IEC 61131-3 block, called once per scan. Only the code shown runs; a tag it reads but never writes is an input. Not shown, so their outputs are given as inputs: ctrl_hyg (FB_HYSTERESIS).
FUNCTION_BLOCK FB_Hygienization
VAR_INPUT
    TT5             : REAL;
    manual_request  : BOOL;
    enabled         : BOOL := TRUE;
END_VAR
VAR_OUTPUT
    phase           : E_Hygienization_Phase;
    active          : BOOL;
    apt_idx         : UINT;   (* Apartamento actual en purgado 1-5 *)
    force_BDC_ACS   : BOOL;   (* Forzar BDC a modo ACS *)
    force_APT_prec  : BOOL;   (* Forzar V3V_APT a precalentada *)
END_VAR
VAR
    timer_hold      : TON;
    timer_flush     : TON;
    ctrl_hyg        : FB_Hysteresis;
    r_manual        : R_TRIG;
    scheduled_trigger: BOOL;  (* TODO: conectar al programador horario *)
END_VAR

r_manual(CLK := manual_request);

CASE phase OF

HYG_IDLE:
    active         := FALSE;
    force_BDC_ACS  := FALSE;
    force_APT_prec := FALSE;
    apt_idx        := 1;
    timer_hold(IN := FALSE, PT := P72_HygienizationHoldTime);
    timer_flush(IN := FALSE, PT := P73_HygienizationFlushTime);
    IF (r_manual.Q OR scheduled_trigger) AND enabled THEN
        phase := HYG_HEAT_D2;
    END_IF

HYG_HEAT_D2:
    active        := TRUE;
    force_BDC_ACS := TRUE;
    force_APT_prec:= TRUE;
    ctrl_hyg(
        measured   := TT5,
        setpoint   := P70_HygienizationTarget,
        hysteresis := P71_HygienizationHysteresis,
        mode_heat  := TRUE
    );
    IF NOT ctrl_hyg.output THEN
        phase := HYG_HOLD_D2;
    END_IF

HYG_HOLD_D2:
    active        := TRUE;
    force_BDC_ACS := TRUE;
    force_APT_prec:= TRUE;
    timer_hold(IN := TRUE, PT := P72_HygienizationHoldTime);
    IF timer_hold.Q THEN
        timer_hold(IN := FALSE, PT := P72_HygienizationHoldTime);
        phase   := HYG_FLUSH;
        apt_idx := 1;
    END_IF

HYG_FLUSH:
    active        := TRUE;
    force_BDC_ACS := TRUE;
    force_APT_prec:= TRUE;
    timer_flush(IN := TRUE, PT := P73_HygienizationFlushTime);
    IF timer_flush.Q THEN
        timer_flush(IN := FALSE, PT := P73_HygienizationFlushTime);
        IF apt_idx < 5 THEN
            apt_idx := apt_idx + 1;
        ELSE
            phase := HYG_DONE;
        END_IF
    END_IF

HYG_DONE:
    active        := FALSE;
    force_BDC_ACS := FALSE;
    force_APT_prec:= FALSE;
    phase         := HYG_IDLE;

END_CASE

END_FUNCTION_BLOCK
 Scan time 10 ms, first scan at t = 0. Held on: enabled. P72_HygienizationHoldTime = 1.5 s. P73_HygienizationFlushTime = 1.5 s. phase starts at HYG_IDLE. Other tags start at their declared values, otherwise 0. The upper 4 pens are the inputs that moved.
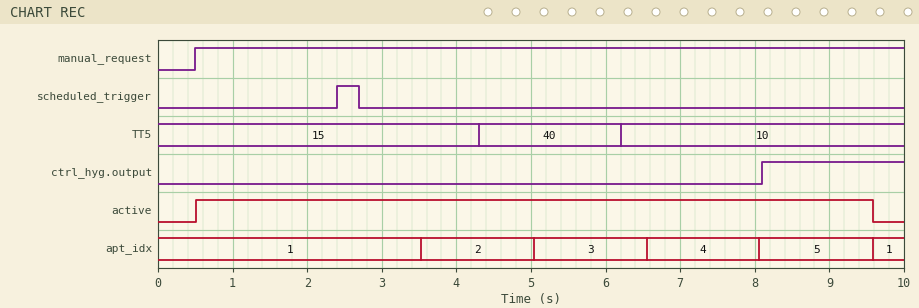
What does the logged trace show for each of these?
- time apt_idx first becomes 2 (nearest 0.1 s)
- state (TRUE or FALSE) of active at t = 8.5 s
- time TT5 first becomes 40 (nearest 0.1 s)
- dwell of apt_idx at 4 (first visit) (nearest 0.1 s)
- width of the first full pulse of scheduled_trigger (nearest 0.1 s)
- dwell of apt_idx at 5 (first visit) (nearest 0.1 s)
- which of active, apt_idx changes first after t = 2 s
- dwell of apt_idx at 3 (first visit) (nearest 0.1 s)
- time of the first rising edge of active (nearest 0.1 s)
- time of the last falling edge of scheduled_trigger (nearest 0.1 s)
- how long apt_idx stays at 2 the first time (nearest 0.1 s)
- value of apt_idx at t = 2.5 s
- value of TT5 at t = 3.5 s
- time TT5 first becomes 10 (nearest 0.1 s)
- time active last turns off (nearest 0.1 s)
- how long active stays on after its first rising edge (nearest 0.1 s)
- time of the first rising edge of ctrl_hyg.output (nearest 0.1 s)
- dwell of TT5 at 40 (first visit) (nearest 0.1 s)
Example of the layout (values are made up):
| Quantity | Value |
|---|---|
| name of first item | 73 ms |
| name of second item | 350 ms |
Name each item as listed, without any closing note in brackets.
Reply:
| Quantity | Value |
|---|---|
| time apt_idx first becomes 2 | 3.5 s |
| state (TRUE or FALSE) of active at t = 8.5 s | TRUE |
| time TT5 first becomes 40 | 4.3 s |
| dwell of apt_idx at 4 (first visit) | 1.5 s |
| width of the first full pulse of scheduled_trigger | 0.3 s |
| dwell of apt_idx at 5 (first visit) | 1.5 s |
| which of active, apt_idx changes first after t = 2 s | apt_idx |
| dwell of apt_idx at 3 (first visit) | 1.5 s |
| time of the first rising edge of active | 0.5 s |
| time of the last falling edge of scheduled_trigger | 2.7 s |
| how long apt_idx stays at 2 the first time | 1.5 s |
| value of apt_idx at t = 2.5 s | 1 |
| value of TT5 at t = 3.5 s | 15 |
| time TT5 first becomes 10 | 6.2 s |
| time active last turns off | 9.6 s |
| how long active stays on after its first rising edge | 9.1 s |
| time of the first rising edge of ctrl_hyg.output | 8.1 s |
| dwell of TT5 at 40 (first visit) | 1.9 s |
